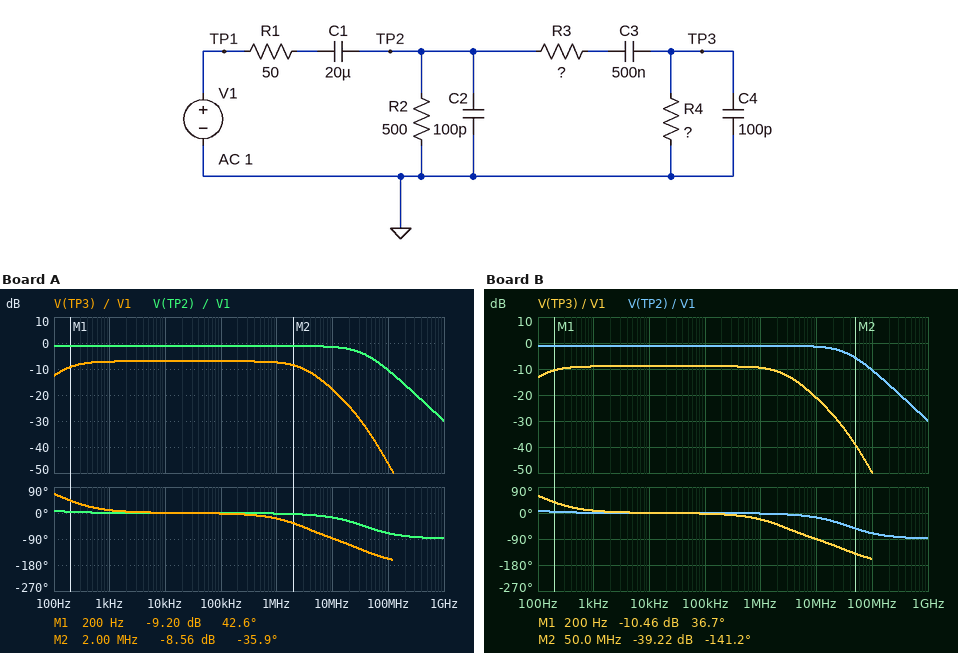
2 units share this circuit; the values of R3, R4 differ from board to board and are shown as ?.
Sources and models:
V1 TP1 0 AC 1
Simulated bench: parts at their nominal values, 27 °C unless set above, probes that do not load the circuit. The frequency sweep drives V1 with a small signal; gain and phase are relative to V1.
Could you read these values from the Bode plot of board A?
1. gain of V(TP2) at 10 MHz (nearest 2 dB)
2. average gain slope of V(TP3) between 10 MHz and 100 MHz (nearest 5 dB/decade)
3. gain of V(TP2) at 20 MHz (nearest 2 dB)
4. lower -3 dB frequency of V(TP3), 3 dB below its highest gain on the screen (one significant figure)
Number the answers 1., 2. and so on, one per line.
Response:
1. -2 dB
2. -30 dB/decade
3. -2 dB
4. 200 Hz
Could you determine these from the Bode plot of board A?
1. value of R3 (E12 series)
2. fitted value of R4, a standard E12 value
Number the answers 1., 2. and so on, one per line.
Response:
1. 1 kΩ
2. 1 kΩ
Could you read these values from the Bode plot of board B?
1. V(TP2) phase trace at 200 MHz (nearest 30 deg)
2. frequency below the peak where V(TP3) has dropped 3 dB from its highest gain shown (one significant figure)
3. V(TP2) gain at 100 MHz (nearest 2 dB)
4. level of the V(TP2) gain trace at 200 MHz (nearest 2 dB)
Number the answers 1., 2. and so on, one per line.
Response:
1. -90 deg
2. 100 Hz
3. -10 dB
4. -16 dB
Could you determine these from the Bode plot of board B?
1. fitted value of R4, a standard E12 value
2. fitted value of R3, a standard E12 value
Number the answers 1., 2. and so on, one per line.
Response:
1. 1 kΩ
2. 1.5 kΩ
